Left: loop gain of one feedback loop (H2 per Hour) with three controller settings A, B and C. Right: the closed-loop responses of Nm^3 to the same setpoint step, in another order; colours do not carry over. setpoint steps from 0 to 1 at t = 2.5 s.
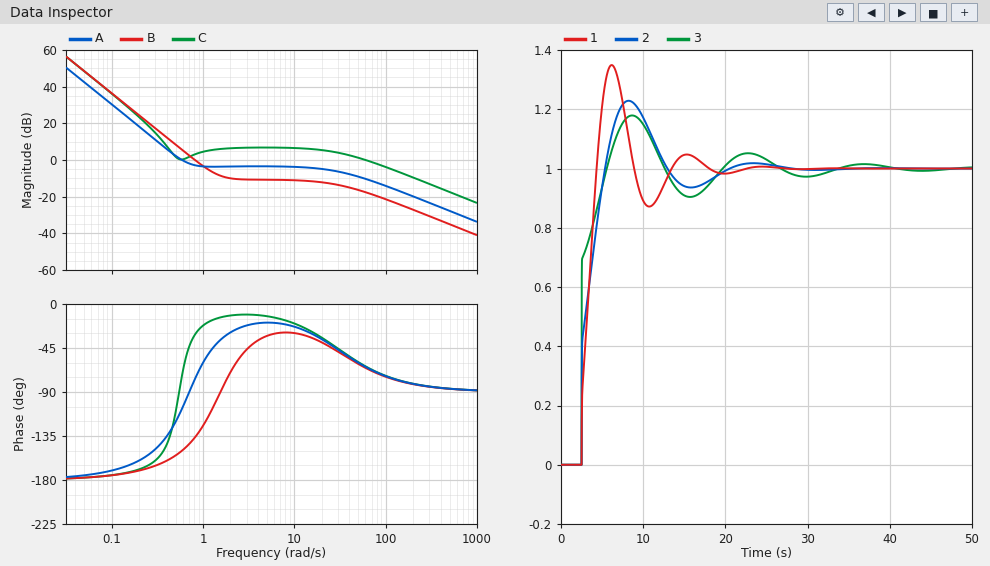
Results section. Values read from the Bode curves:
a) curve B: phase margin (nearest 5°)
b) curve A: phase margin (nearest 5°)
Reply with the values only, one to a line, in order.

45°
75°
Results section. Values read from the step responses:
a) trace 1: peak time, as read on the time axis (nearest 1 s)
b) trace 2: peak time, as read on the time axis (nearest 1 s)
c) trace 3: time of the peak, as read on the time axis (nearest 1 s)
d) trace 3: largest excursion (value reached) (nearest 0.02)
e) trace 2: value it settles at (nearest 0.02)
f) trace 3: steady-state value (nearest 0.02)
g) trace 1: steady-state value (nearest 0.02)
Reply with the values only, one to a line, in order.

6 s
8 s
9 s
1.18
1.00
1.00
1.00
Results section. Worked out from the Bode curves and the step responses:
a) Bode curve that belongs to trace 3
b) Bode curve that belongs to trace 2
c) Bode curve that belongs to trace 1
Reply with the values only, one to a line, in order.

C
A
B
